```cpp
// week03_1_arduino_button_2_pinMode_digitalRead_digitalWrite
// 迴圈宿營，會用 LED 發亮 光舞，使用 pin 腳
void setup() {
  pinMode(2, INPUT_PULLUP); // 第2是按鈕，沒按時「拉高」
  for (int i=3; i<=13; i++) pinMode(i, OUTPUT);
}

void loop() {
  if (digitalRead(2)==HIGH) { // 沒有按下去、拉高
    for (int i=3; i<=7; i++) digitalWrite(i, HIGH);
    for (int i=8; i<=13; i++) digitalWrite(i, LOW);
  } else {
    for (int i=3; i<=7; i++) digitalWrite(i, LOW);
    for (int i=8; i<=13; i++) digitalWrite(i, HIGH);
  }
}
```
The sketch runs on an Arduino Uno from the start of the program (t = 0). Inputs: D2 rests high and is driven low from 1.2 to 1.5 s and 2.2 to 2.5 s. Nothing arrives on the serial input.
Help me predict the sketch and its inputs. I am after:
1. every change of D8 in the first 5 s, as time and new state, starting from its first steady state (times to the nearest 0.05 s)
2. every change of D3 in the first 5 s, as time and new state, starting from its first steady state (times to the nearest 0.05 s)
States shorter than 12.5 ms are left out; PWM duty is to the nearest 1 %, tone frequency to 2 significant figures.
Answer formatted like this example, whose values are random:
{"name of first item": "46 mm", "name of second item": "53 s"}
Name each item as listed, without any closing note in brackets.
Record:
{"every change of D8 in the first 5 s, as time and new state, starting from its first steady state": "0 s low; 1.2 s high; 1.5 s low; 2.2 s high; 2.5 s low", "every change of D3 in the first 5 s, as time and new state, starting from its first steady state": "0 s high; 1.2 s low; 1.5 s high; 2.2 s low; 2.5 s high"}
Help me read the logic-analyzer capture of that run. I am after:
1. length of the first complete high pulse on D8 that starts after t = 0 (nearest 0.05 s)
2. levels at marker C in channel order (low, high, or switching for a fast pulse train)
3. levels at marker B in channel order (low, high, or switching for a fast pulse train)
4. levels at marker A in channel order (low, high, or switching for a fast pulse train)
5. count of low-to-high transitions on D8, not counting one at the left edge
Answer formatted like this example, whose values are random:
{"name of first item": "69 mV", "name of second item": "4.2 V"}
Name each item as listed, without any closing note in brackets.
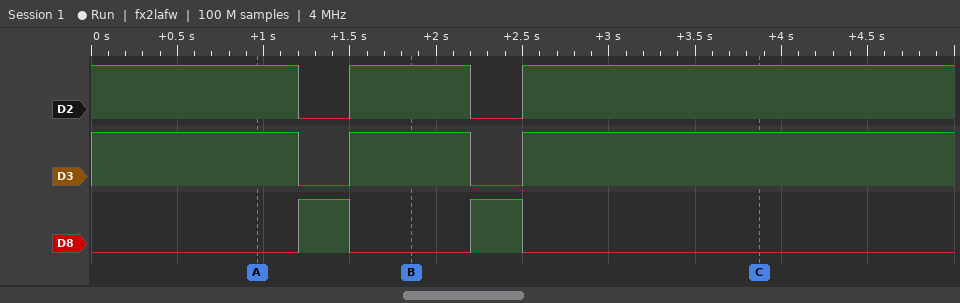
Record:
{"length of the first complete high pulse on D8 that starts after t = 0": "0.30 s", "levels at marker C in channel order": "D2 high, D3 high, D8 low", "levels at marker B in channel order": "D2 high, D3 high, D8 low", "levels at marker A in channel order": "D2 high, D3 high, D8 low", "count of low-to-high transitions on D8, not counting one at the left edge": "2"}
